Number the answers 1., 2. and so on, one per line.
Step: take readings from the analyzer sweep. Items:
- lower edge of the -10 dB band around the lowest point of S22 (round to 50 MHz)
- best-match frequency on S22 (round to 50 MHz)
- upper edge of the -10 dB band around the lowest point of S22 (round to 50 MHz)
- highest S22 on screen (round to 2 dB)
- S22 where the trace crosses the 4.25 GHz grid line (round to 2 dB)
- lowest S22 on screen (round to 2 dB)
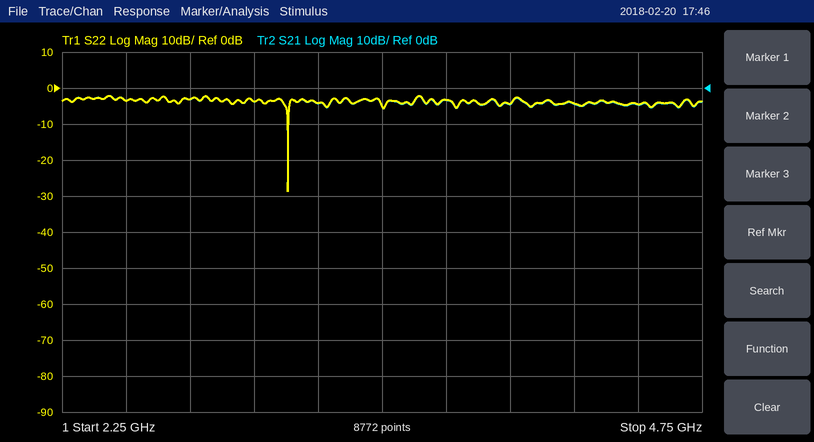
1. 3.15 GHz
2. 3.15 GHz
3. 3.15 GHz
4. -2 dB
5. -4 dB
6. -28 dB
